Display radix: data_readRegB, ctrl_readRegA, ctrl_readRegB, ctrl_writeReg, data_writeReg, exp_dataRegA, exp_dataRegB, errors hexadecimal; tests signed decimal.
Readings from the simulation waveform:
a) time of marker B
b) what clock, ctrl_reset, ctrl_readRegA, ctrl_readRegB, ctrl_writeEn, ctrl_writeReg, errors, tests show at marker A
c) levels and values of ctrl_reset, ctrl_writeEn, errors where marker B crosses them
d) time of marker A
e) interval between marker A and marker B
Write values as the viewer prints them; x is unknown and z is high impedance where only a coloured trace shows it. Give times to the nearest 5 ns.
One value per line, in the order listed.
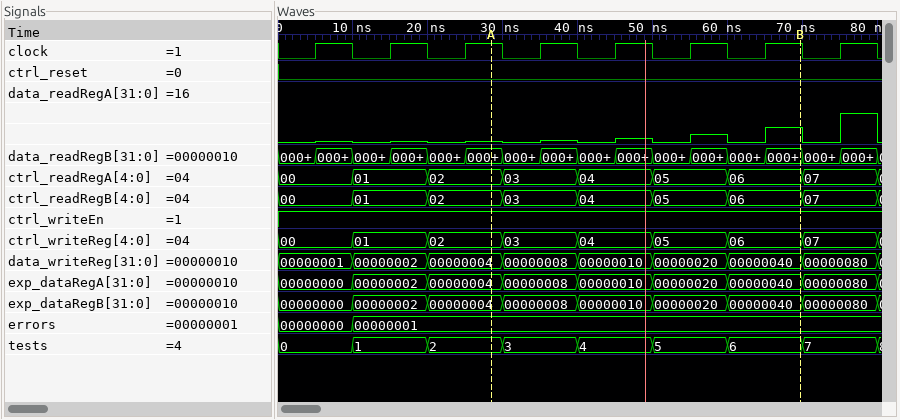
70 ns
clock=1, ctrl_reset=0, ctrl_readRegA=02, ctrl_readRegB=02, ctrl_writeEn=1, ctrl_writeReg=02, errors=00000001, tests=2
ctrl_reset=0, ctrl_writeEn=1, errors=00000001
30 ns
40 ns
